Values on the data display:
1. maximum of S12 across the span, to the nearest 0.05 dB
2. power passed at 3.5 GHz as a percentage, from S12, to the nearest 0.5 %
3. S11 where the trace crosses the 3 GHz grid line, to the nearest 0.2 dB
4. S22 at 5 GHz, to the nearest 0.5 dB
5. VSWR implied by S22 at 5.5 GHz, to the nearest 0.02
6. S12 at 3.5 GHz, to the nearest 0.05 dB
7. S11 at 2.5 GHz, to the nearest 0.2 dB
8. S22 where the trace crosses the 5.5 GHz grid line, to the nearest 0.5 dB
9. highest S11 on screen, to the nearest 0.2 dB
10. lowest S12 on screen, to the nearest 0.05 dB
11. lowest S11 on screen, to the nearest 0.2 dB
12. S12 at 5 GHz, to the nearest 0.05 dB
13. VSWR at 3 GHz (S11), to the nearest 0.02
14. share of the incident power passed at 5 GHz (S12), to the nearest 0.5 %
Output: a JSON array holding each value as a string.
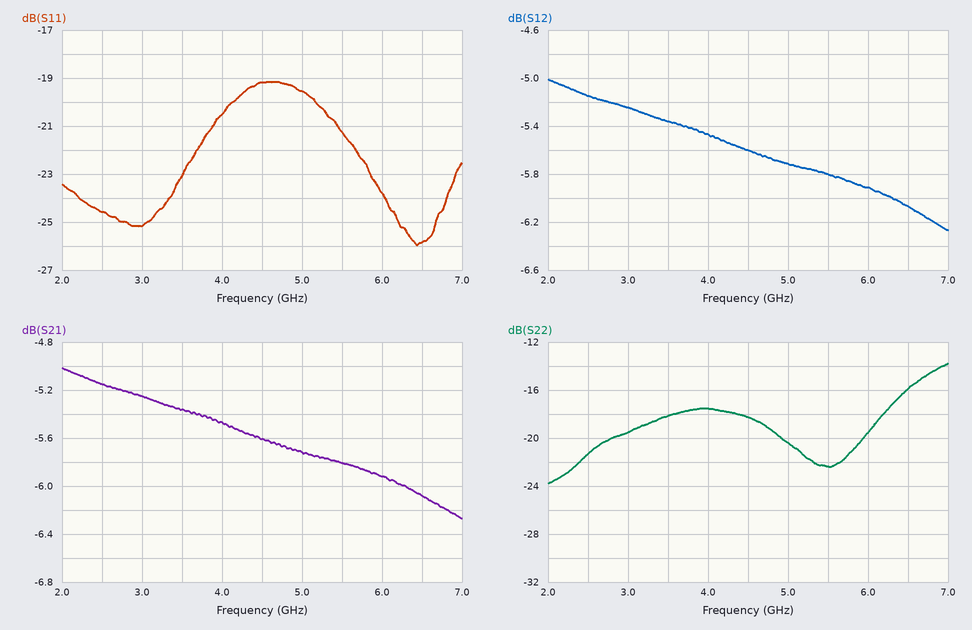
["-5.00 dB", "29.0 %", "-25.2 dB", "-20.5 dB", "1.16", "-5.35 dB", "-24.6 dB", "-22.5 dB", "-19.2 dB", "-6.25 dB", "-26.0 dB", "-5.70 dB", "1.12", "27.0 %"]
